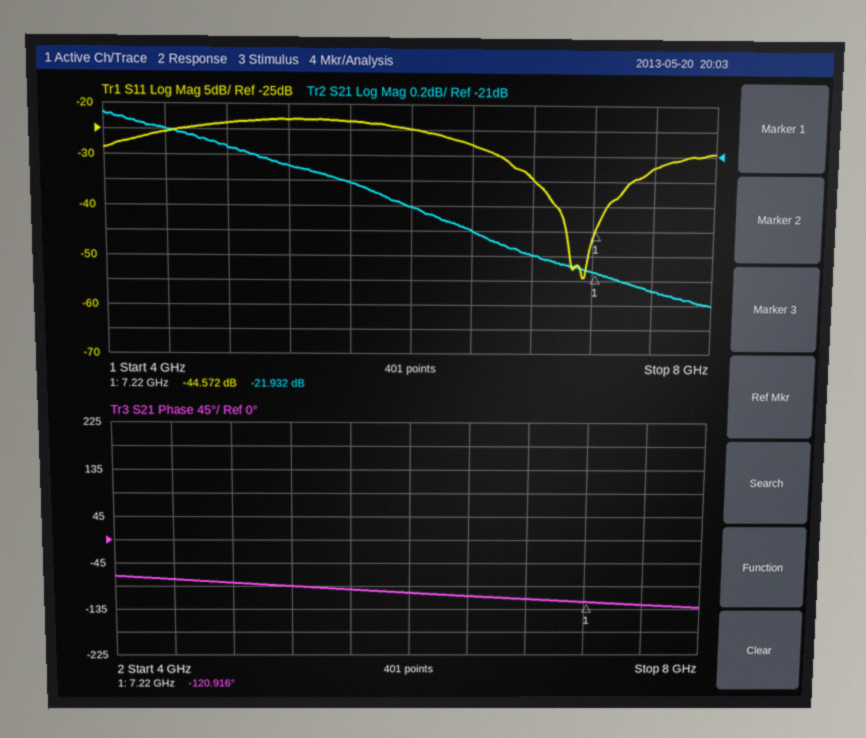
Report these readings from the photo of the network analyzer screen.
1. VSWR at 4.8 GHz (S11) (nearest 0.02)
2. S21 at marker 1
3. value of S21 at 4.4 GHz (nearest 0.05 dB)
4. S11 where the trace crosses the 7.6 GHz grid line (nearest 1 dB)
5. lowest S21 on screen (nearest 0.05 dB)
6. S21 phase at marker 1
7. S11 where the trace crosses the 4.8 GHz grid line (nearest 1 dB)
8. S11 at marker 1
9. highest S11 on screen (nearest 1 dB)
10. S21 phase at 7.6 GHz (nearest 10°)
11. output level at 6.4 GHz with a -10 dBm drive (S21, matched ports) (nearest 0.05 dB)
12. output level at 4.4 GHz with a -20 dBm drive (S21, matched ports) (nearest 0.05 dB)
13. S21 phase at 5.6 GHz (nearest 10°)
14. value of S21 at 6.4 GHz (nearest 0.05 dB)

1.14
-21.932 dB
-20.80 dB
-32 dB
-22.20 dB
-120.916°
-24 dB
-44.572 dB
-23 dB
-130°
-31.60 dBm
-40.80 dBm
-100°
-21.60 dB
